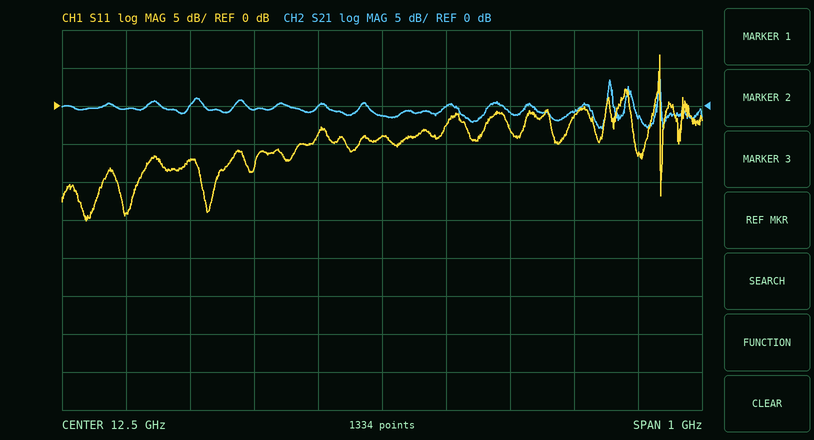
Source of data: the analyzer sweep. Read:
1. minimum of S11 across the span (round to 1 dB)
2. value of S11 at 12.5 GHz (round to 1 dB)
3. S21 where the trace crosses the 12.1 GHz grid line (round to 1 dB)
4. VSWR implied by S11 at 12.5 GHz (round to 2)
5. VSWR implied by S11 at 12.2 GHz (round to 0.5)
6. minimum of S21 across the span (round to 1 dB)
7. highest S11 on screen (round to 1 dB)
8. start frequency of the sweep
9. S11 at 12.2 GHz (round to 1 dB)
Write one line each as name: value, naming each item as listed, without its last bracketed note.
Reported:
minimum of S11 across the span: -15 dB
value of S11 at 12.5 GHz: -4 dB
S21 where the trace crosses the 12.1 GHz grid line: 0 dB
VSWR implied by S11 at 12.5 GHz: 4
VSWR implied by S11 at 12.2 GHz: 2.5
minimum of S21 across the span: -3 dB
highest S11 on screen: 7 dB
start frequency of the sweep: 12 GHz
S11 at 12.2 GHz: -7 dB
